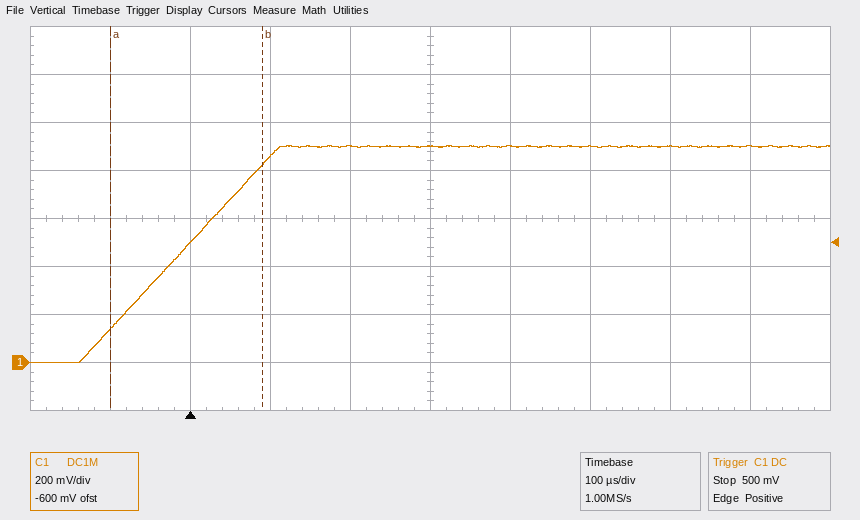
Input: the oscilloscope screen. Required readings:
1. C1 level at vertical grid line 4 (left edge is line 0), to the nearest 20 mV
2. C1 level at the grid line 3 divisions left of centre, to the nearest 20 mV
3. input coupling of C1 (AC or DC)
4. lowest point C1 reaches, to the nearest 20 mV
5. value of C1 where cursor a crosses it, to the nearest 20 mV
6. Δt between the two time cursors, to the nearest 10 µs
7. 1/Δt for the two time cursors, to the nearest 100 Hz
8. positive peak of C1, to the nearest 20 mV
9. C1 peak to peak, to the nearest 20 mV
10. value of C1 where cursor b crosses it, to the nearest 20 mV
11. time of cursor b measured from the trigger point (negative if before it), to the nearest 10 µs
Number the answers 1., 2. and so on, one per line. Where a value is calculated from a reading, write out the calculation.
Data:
1. 900 mV
2. 500 mV
3. DC
4. 0 mV
5. 140 mV
6. 190 µs
7. 1 / 190 µs ≈ 5.3 kHz
8. 900 mV
9. 900 mV − (0 mV) = 900 mV
10. 820 mV
11. +90 µs
